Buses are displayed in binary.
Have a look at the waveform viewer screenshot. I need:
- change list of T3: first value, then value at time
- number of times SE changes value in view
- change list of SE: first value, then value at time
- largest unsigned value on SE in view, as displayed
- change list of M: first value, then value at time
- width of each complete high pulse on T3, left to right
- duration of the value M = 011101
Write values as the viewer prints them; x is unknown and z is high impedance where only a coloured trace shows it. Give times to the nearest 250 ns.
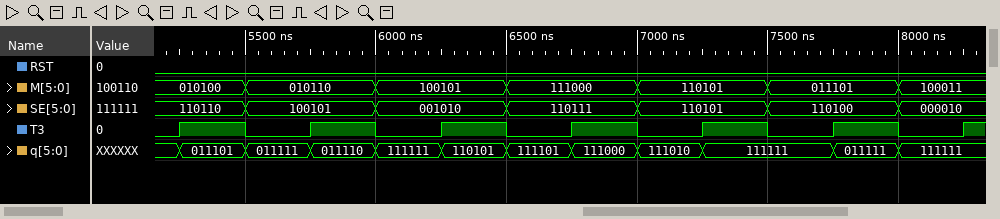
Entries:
0, 1 at 5250 ns, 0 at 5500 ns, 1 at 5750 ns, 0 at 6000 ns, 1 at 6250 ns, 0 at 6500 ns, 1 at 6750 ns, 0 at 7000 ns, 1 at 7250 ns, 0 at 7500 ns, 1 at 7750 ns, 0 at 8000 ns, 1 at 8250 ns
6
110110, 100101 at 5500 ns, 001010 at 6000 ns, 110111 at 6500 ns, 110101 at 7000 ns, 110100 at 7500 ns, 000010 at 8000 ns
110111
010100, 010110 at 5500 ns, 100101 at 6000 ns, 111000 at 6500 ns, 110101 at 7000 ns, 011101 at 7500 ns, 100011 at 8000 ns
250 ns, 250 ns, 250 ns, 250 ns, 250 ns, 250 ns
500 ns
